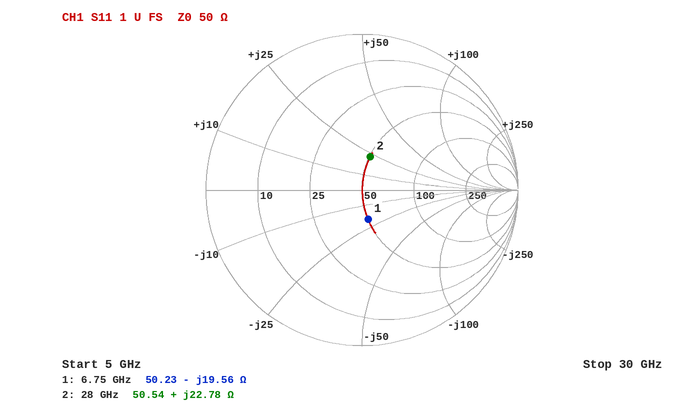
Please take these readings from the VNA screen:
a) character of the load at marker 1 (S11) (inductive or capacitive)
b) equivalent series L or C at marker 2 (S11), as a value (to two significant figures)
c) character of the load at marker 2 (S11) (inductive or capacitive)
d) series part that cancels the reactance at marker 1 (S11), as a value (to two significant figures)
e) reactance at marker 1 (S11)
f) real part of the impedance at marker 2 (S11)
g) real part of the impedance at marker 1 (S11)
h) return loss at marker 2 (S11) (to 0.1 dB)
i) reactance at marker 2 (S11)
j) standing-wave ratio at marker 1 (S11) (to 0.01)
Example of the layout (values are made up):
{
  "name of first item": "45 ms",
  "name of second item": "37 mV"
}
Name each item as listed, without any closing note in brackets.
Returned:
{
  "character of the load at marker 1 (S11)": "capacitive",
  "equivalent series L or C at marker 2 (S11), as a value": "130 pH",
  "character of the load at marker 2 (S11)": "inductive",
  "series part that cancels the reactance at marker 1 (S11), as a value": "460 pH",
  "reactance at marker 1": "-19.56 Ω",
  "real part of the impedance at marker 2": "50.54 Ω",
  "real part of the impedance at marker 1": "50.23 Ω",
  "return loss at marker 2 (S11)": "13.1 dB",
  "reactance at marker 2": "+22.78 Ω",
  "standing-wave ratio at marker 1 (S11)": "1.47"
}
